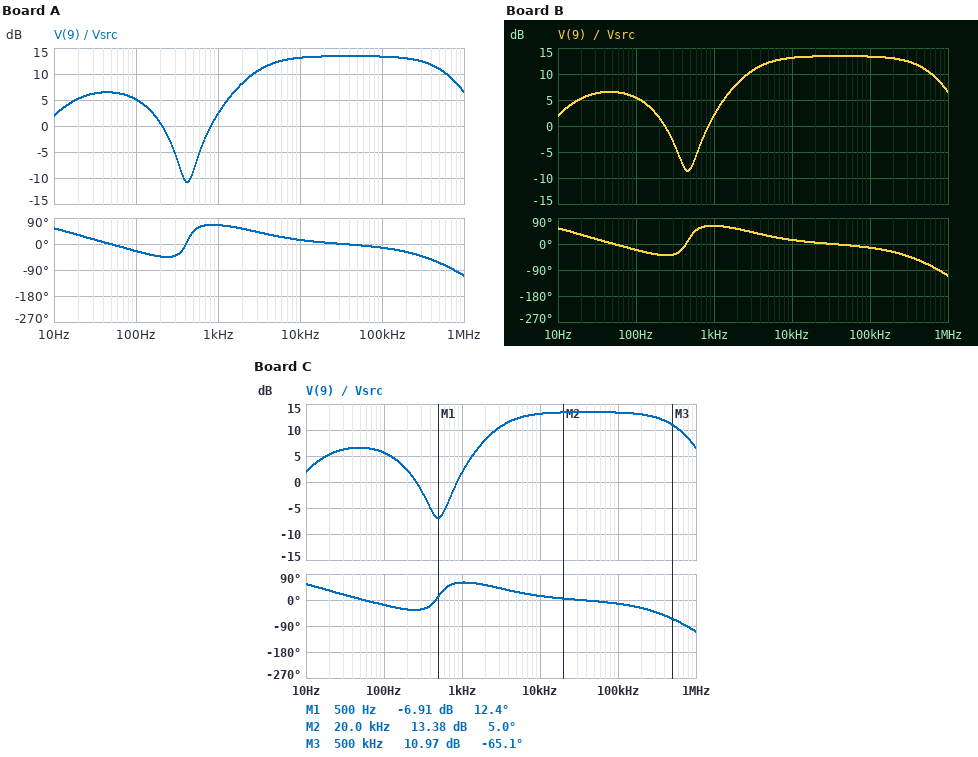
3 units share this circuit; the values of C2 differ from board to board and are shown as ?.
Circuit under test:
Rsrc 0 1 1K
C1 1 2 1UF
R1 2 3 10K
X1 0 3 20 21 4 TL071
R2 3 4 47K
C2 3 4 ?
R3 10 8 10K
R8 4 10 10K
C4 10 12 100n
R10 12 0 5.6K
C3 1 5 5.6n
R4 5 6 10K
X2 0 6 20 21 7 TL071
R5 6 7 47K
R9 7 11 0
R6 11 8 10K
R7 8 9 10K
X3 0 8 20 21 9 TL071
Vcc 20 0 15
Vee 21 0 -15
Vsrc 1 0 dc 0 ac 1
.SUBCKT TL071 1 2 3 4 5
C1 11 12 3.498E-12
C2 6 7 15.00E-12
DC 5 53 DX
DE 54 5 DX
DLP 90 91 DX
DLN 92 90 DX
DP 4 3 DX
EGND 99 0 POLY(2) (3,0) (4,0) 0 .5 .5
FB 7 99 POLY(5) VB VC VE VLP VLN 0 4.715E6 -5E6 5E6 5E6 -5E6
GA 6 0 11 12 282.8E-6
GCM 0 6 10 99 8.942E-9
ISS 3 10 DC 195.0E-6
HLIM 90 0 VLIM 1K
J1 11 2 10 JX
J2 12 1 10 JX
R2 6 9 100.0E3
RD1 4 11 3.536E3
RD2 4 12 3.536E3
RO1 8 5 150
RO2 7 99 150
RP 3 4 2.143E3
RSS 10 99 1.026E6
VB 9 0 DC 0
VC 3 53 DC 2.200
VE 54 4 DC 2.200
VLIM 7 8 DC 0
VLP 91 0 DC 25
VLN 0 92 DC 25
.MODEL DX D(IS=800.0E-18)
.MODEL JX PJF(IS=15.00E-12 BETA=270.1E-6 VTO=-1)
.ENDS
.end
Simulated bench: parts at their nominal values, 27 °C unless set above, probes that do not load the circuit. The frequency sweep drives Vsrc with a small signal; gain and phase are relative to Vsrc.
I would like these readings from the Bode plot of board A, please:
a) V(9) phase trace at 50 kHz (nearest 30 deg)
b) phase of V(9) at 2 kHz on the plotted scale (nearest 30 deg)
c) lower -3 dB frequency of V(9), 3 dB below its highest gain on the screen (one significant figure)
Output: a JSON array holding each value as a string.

["0 deg", "60 deg", "3 kHz"]
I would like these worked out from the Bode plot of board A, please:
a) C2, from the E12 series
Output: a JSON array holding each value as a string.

["15 nF"]
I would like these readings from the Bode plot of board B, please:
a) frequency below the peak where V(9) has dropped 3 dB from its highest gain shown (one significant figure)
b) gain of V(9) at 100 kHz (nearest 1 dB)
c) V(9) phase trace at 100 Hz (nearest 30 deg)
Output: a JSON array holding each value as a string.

["3 kHz", "13 dB", "-30 deg"]
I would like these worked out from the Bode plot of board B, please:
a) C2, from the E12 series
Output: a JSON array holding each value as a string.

["12 nF"]
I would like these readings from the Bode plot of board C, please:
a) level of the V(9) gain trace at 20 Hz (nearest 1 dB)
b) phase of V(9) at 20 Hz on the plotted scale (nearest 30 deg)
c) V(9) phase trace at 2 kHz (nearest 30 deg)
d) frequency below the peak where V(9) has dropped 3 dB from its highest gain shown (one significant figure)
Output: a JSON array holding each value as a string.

["5 dB", "30 deg", "60 deg", "3 kHz"]
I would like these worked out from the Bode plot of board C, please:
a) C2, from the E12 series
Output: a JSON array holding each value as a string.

["10 nF"]
